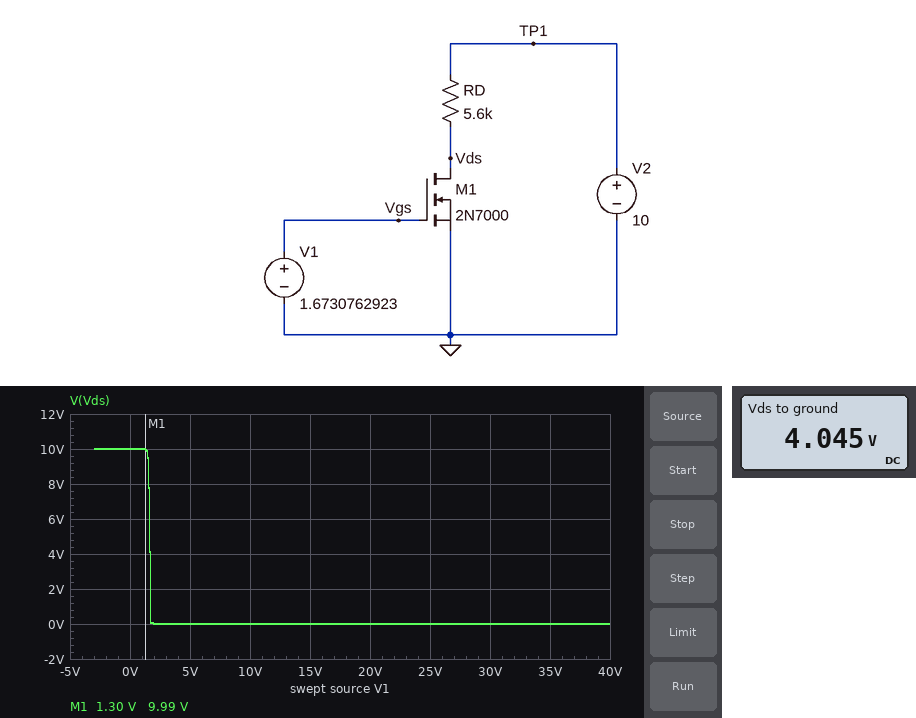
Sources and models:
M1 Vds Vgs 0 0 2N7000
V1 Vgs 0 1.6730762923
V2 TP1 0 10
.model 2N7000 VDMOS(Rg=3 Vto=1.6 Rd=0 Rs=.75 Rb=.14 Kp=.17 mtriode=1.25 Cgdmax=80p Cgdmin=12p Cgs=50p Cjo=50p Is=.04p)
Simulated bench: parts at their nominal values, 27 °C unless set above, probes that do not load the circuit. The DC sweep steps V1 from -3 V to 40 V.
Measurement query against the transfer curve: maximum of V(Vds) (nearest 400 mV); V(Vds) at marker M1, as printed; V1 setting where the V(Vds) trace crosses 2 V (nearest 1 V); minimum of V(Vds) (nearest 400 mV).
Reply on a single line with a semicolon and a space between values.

10.0 V; 9.99 V; 2 V; 0 V
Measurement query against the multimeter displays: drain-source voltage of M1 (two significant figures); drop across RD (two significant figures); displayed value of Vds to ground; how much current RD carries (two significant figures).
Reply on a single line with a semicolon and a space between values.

4.0 V; 6.0 V; 4.045 V; 1.1 mA
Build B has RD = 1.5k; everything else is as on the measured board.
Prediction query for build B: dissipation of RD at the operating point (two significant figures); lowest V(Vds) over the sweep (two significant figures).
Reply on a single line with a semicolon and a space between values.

1.7 mW; 5.8 mV
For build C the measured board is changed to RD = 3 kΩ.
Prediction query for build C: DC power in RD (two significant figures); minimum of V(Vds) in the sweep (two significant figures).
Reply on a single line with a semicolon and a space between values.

3.4 mW; 2.9 mV
